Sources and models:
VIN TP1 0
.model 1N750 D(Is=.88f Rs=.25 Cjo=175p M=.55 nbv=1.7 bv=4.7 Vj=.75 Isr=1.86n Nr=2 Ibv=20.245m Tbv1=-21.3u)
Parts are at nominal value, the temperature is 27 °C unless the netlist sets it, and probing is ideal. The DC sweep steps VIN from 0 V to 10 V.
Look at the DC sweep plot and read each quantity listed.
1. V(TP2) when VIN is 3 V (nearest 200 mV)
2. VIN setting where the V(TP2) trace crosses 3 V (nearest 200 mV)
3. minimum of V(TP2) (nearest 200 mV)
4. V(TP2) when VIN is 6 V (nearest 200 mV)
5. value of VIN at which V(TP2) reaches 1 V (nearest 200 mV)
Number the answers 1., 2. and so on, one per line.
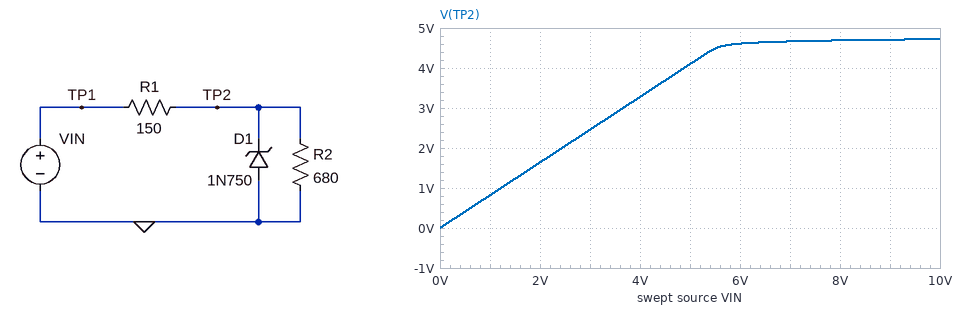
1. 2.4 V
2. 3.6 V
3. 0 V
4. 4.6 V
5. 1.2 V
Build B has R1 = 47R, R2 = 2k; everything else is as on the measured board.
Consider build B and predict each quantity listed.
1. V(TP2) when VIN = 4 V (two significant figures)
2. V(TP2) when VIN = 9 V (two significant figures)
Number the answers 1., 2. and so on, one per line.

1. 3.9 V
2. 4.8 V
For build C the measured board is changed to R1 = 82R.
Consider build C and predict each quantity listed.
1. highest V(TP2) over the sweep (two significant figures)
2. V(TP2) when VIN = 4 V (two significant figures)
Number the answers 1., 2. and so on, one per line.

1. 4.8 V
2. 3.6 V
